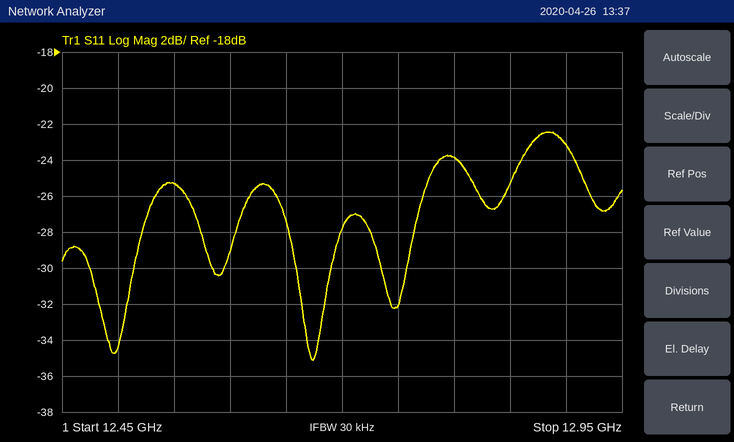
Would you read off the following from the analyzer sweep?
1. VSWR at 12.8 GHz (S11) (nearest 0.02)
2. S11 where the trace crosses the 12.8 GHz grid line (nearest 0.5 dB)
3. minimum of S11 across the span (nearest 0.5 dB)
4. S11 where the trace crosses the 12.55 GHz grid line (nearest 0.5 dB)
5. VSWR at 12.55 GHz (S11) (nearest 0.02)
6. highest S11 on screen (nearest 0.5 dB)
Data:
1.14
-24.0 dB
-35.0 dB
-25.5 dB
1.12
-22.5 dB
